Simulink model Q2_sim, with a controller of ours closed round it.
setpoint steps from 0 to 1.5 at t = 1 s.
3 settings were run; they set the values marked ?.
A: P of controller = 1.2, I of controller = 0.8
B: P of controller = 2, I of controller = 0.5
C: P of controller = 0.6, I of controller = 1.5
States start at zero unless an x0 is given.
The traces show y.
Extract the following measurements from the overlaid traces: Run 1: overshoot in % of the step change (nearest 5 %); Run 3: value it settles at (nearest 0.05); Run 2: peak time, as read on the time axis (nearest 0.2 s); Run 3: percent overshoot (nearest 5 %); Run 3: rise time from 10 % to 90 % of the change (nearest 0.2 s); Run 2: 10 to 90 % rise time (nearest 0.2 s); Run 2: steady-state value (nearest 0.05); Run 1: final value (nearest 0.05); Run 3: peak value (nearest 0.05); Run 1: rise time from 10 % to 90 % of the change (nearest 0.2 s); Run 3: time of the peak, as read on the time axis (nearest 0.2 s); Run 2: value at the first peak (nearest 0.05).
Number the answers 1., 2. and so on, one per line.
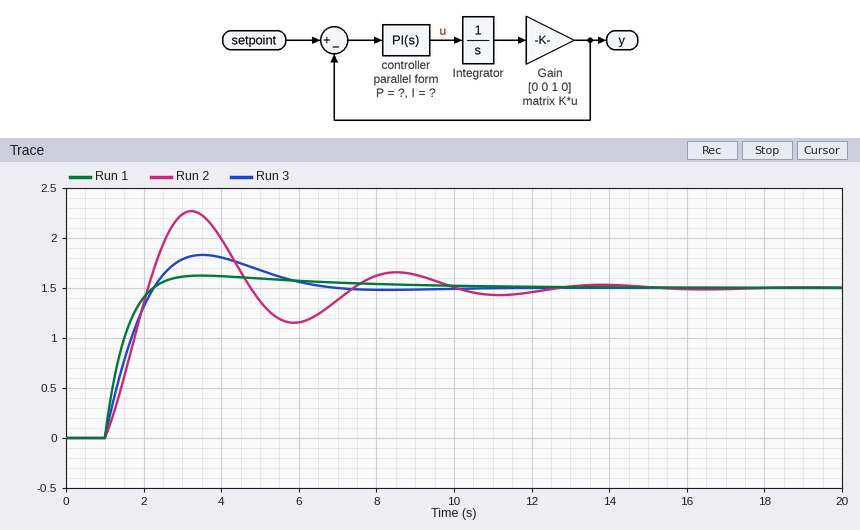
1. 10 %
2. 1.50
3. 3.2 s
4. 20 %
5. 1.0 s
6. 0.8 s
7. 1.50
8. 1.50
9. 1.85
10. 0.8 s
11. 3.6 s
12. 2.25
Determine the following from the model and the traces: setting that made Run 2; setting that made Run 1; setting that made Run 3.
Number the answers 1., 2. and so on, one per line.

1. C
2. B
3. A
